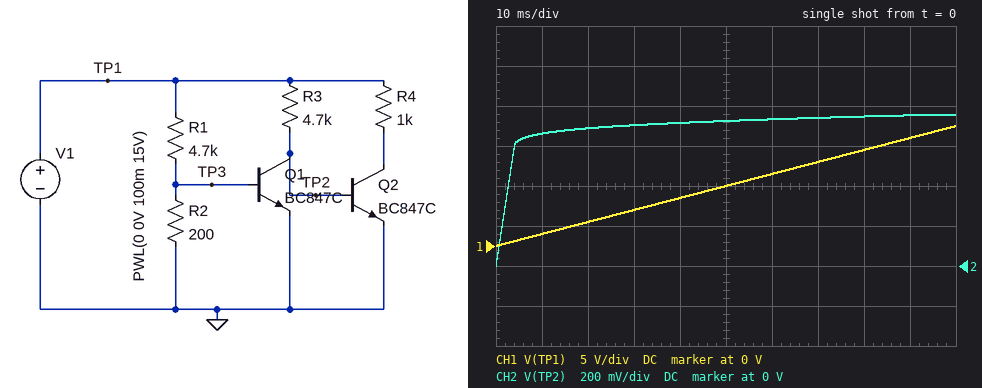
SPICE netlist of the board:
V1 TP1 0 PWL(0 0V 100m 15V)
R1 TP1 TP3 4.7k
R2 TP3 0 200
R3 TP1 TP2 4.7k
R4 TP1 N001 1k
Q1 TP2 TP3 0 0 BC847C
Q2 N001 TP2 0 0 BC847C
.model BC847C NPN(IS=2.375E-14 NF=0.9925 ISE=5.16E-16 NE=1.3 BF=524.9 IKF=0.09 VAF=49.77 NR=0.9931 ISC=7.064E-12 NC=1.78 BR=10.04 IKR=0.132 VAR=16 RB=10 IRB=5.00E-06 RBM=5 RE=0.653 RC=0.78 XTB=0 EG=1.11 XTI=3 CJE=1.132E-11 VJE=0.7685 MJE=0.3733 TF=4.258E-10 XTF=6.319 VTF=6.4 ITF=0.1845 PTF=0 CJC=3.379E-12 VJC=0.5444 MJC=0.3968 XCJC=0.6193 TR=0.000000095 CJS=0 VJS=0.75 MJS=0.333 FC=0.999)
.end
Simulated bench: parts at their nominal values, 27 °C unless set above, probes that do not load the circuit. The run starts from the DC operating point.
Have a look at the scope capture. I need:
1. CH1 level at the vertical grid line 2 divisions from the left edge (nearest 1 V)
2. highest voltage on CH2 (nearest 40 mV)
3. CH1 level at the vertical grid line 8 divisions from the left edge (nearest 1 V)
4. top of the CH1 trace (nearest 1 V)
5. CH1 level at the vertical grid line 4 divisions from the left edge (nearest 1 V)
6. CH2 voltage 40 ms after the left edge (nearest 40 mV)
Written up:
3 V
760 mV
12 V
15 V
6 V
720 mV
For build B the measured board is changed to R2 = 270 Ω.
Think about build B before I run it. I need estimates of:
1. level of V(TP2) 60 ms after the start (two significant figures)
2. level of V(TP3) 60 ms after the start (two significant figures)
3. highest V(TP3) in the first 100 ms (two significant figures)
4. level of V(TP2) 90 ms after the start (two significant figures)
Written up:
730 mV
490 mV
690 mV
29 mV
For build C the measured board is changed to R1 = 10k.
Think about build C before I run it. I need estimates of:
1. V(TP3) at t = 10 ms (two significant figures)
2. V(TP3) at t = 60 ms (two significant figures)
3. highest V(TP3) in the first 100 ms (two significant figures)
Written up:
29 mV
180 mV
290 mV
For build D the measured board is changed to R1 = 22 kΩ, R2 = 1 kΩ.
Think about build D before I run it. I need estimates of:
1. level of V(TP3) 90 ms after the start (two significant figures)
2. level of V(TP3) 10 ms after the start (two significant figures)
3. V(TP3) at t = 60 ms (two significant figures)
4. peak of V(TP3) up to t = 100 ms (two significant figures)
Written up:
590 mV
65 mV
390 mV
650 mV
